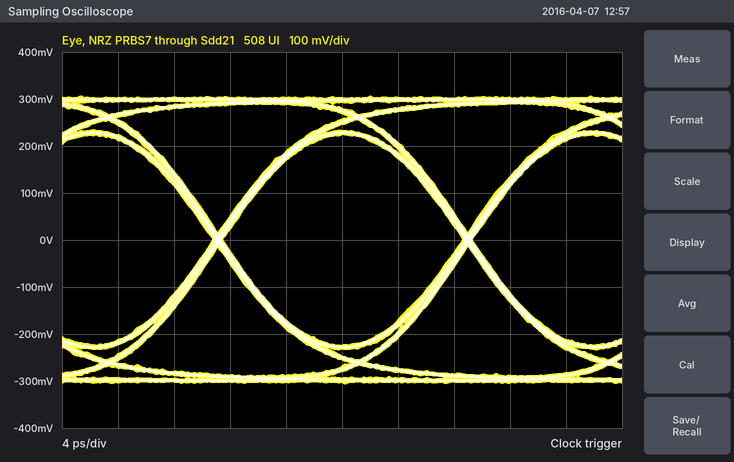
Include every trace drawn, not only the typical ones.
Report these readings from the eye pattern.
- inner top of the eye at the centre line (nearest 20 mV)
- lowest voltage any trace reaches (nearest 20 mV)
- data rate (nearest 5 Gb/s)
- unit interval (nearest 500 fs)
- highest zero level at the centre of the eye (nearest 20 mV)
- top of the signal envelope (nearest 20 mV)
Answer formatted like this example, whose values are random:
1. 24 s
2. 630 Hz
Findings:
1. 220 mV
2. -300 mV
3. 55 Gb/s
4. 18.0 ps
5. -220 mV
6. 300 mV
